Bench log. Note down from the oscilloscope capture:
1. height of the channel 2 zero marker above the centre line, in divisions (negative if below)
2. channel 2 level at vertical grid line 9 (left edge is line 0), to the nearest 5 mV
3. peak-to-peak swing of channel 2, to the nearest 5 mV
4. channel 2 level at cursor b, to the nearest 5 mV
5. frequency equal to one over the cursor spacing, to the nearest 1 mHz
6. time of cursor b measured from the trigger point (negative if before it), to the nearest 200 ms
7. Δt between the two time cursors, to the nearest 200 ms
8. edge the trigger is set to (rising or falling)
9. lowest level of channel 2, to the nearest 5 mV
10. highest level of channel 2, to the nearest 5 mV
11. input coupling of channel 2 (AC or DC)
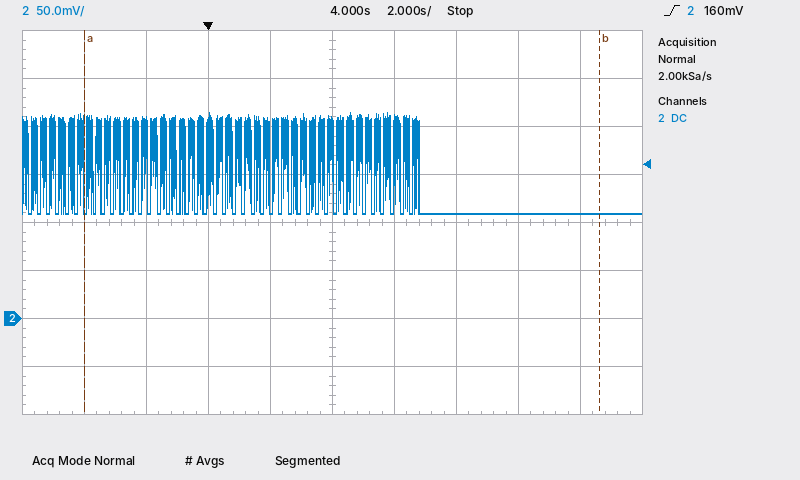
-2.0 div
110 mV
105 mV
110 mV
60 mHz
+12.6 s
16.6 s
rising
110 mV
215 mV
DC
